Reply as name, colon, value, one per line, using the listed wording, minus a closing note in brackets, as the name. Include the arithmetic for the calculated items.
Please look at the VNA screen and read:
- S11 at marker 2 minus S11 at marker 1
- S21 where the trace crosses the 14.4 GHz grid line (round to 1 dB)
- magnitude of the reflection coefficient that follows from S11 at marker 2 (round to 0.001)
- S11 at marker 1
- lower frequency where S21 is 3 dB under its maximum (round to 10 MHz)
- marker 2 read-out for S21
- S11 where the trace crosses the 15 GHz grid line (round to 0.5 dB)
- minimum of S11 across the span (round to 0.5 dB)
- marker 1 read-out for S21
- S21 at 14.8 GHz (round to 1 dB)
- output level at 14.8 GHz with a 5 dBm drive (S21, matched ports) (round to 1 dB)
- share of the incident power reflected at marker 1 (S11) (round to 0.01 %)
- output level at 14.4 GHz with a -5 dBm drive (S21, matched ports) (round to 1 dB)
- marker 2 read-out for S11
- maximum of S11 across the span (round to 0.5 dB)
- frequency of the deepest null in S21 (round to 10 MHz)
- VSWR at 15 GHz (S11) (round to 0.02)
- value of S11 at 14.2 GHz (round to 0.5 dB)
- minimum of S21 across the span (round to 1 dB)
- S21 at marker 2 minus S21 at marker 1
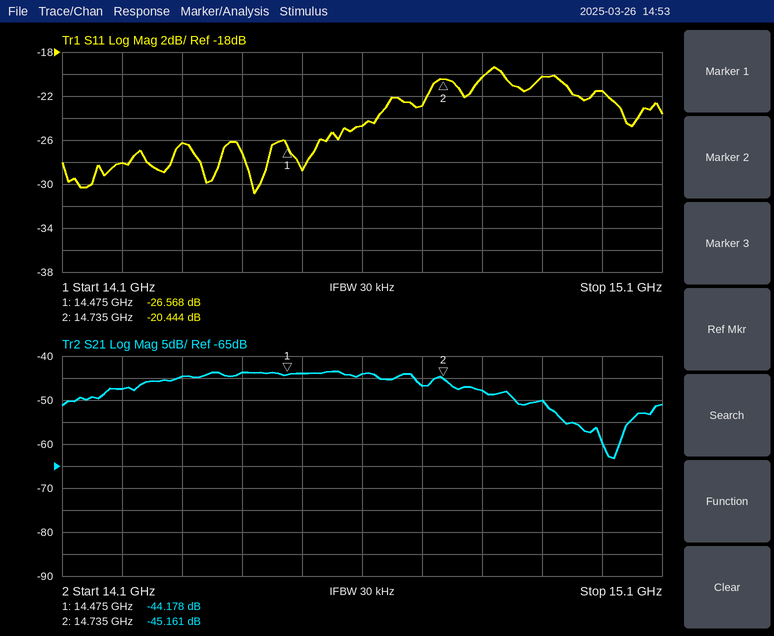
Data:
S11 at marker 2 minus S11 at marker 1: -20.444 − (-26.568) = 6.124 dB
S21 where the trace crosses the 14.4 GHz grid line: -44 dB
magnitude of the reflection coefficient that follows from S11 at marker 2: 10^(-20.444/20) ≈ 0.095
S11 at marker 1: -26.568 dB
lower frequency where S21 is 3 dB under its maximum: 14.23 GHz
marker 2 read-out for S21: -45.161 dB
S11 where the trace crosses the 15 GHz grid line: -21.5 dB
minimum of S11 across the span: -31.0 dB
marker 1 read-out for S21: -44.178 dB
S21 at 14.8 GHz: -48 dB
output level at 14.8 GHz with a 5 dBm drive (S21, matched ports): 5 dBm + (-48 dB) = -43 dBm
share of the incident power reflected at marker 1 (S11): 10^(-26.568/10) ≈ 0.22 %
output level at 14.4 GHz with a -5 dBm drive (S21, matched ports): -5 dBm + (-44 dB) = -49 dBm
marker 2 read-out for S11: -20.444 dB
maximum of S11 across the span: -19.5 dB
frequency of the deepest null in S21: 15.02 GHz
VSWR at 15 GHz (S11): |Γ| = 10^(-21.5/20) = 0.0841; VSWR = (1 + 0.0841)/(1 − 0.0841) ≈ 1.18
value of S11 at 14.2 GHz: -28.0 dB
minimum of S21 across the span: -63 dB
S21 at marker 2 minus S21 at marker 1: -45.161 − (-44.178) = -0.983 dB
